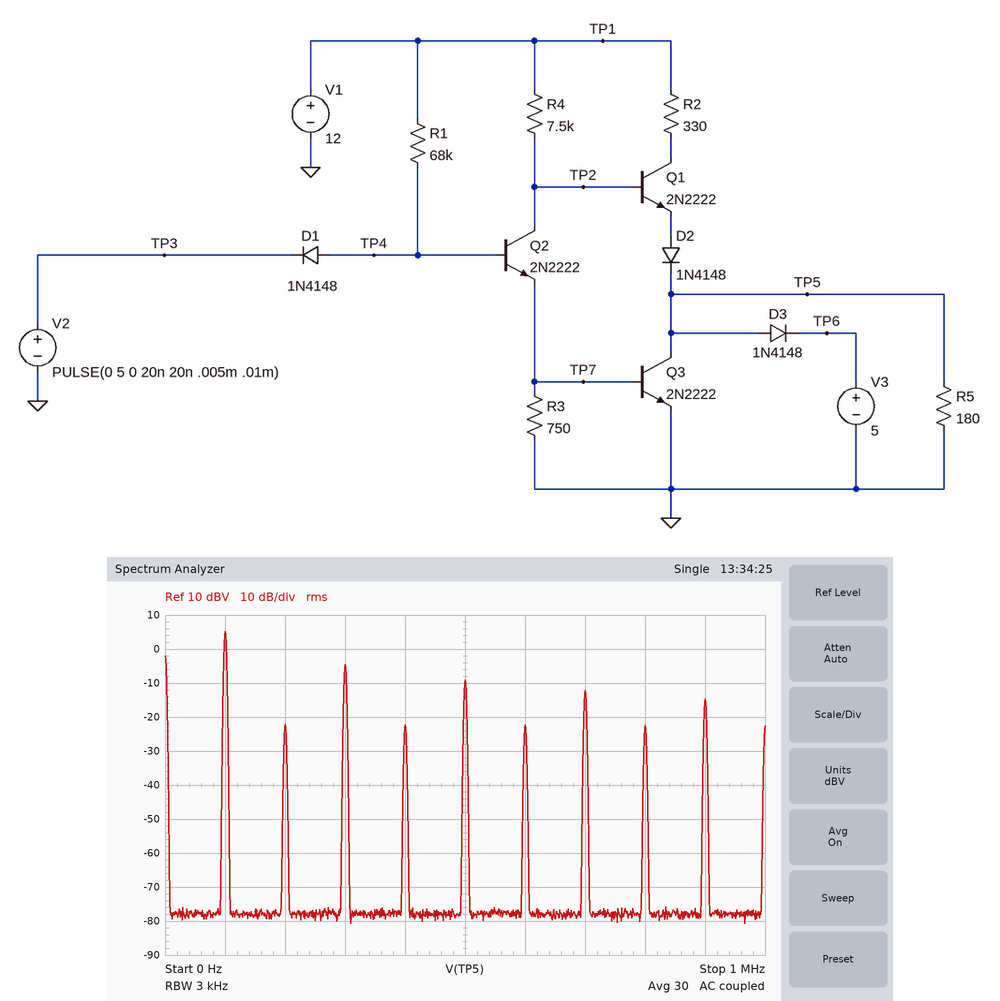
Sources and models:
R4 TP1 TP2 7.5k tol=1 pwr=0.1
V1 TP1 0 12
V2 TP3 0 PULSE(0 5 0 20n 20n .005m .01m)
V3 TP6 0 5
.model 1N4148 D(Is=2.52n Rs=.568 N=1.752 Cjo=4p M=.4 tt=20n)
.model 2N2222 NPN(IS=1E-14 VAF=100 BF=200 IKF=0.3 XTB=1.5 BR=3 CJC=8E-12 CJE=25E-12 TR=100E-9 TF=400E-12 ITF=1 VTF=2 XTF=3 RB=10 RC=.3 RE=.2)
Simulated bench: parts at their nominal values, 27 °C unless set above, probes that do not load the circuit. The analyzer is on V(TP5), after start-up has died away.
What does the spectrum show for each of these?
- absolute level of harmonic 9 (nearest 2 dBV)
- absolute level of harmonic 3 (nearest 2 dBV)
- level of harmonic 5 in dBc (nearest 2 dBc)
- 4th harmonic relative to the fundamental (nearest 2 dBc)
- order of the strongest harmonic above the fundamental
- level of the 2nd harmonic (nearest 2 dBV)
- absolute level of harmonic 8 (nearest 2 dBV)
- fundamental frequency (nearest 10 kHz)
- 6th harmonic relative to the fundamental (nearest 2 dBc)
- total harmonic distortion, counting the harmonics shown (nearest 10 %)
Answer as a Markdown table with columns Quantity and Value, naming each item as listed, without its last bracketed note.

| Quantity | Value |
|---|---|
| absolute level of harmonic 9 | -14 dBV |
| absolute level of harmonic 3 | -4 dBV |
| level of harmonic 5 in dBc | -14 dBc |
| 4th harmonic relative to the fundamental | -28 dBc |
| order of the strongest harmonic above the fundamental | 3 |
| level of the 2nd harmonic | -22 dBV |
| absolute level of harmonic 8 | -22 dBV |
| fundamental frequency | 100 kHz |
| 6th harmonic relative to the fundamental | -28 dBc |
| total harmonic distortion, counting the harmonics shown | 40 % |
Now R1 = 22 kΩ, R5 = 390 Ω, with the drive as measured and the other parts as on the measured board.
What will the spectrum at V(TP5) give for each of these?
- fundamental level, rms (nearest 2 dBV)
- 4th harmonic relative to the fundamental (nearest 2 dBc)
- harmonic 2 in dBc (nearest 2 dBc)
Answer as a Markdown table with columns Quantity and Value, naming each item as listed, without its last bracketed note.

| Quantity | Value |
|---|---|
| fundamental level, rms | 8 dBV |
| 4th harmonic relative to the fundamental | -24 dBc |
| harmonic 2 in dBc | -24 dBc |
